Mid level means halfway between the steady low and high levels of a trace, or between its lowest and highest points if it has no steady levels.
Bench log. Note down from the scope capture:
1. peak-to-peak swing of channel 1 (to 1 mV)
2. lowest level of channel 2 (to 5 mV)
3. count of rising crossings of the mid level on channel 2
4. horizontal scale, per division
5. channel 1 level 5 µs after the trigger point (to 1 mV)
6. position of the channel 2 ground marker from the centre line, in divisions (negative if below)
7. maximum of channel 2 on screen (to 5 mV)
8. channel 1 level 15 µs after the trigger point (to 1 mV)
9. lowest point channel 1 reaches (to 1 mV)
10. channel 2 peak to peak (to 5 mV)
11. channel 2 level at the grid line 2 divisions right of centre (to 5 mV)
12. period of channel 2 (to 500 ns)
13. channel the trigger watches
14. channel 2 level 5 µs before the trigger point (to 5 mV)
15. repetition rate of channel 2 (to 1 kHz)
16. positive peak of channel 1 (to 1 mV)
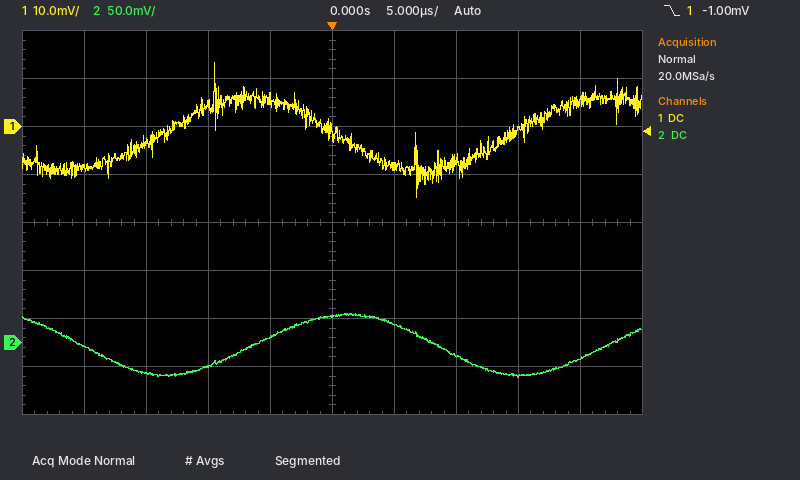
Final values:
28 mV
-35 mV
2
5 µs
-8 mV
-2.5 div
30 mV
-1 mV
-15 mV
65 mV
-15 mV
28.5 µs
channel 1
5 mV
35 kHz
13 mV
